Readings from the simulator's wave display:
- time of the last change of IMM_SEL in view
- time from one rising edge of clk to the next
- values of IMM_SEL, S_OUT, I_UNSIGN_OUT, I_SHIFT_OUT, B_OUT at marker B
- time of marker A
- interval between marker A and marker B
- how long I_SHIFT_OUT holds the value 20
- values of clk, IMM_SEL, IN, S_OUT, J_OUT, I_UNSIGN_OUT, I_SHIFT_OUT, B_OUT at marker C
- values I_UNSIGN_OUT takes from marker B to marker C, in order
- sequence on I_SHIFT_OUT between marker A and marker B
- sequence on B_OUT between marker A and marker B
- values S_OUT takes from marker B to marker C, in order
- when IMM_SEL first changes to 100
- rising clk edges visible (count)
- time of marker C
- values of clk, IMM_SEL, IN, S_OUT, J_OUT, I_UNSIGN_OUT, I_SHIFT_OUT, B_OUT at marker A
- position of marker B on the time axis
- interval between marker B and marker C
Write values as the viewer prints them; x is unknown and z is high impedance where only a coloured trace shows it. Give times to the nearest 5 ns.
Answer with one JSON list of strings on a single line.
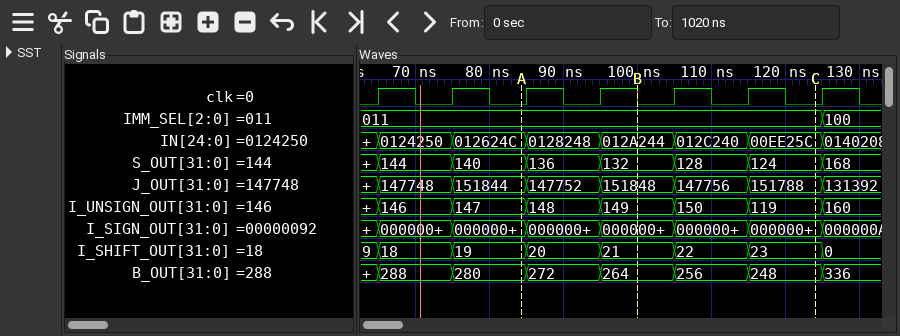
["125 ns", "10 ns", "IMM_SEL=011, S_OUT=132, I_UNSIGN_OUT=149, I_SHIFT_OUT=21, B_OUT=264", "85 ns", "15 ns", "10 ns", "clk=0, IMM_SEL=011, IN=00EE25C, S_OUT=124, J_OUT=151788, I_UNSIGN_OUT=119, I_SHIFT_OUT=23, B_OUT=248", "149, 150, 119", "19, 20, 21", "280, 272, 264", "132, 128, 124", "125 ns", "7", "125 ns", "clk=0, IMM_SEL=011, IN=012624C, S_OUT=140, J_OUT=151844, I_UNSIGN_OUT=147, I_SHIFT_OUT=19, B_OUT=280", "100 ns", "25 ns"]
